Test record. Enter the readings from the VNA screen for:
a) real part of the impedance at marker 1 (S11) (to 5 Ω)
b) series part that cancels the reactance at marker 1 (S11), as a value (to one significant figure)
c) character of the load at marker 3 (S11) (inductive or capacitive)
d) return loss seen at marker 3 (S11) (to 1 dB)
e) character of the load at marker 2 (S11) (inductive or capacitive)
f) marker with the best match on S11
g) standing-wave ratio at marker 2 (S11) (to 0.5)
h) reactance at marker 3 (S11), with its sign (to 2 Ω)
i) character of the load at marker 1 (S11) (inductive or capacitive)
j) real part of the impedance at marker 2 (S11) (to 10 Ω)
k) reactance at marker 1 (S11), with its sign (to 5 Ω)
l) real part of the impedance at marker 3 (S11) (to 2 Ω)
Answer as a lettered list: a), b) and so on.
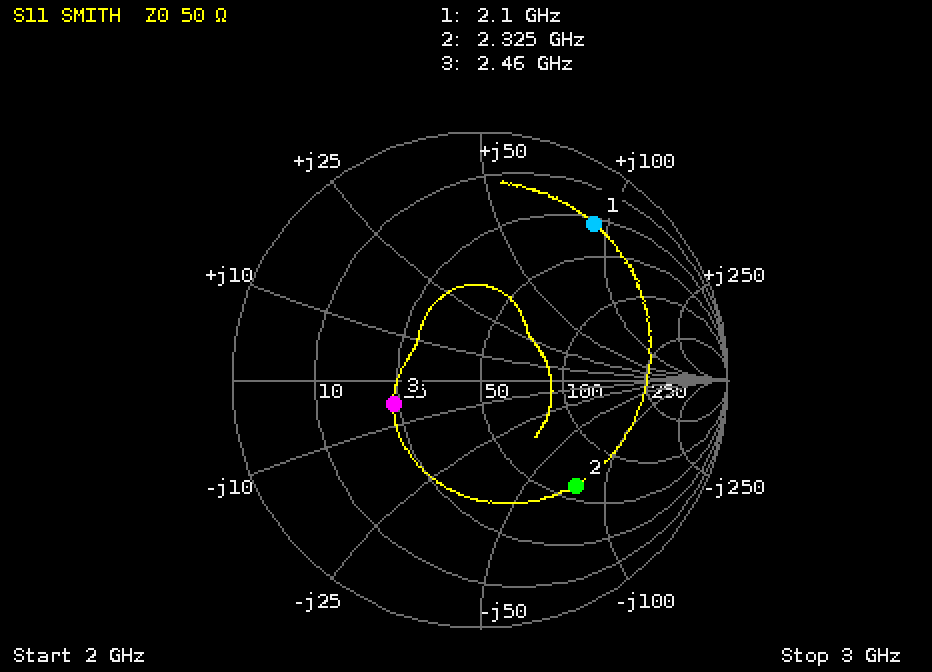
a) 30 Ω
b) 800 fF
c) capacitive
d) 9 dB
e) capacitive
f) marker 3
g) 3.5
h) -6 Ω
i) inductive
j) 60 Ω
k) +90 Ω
l) 24 Ω
